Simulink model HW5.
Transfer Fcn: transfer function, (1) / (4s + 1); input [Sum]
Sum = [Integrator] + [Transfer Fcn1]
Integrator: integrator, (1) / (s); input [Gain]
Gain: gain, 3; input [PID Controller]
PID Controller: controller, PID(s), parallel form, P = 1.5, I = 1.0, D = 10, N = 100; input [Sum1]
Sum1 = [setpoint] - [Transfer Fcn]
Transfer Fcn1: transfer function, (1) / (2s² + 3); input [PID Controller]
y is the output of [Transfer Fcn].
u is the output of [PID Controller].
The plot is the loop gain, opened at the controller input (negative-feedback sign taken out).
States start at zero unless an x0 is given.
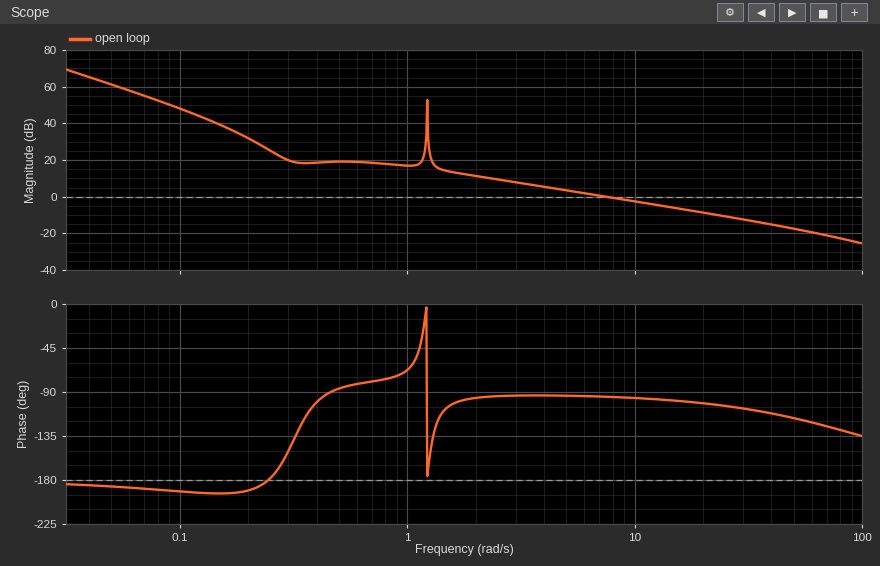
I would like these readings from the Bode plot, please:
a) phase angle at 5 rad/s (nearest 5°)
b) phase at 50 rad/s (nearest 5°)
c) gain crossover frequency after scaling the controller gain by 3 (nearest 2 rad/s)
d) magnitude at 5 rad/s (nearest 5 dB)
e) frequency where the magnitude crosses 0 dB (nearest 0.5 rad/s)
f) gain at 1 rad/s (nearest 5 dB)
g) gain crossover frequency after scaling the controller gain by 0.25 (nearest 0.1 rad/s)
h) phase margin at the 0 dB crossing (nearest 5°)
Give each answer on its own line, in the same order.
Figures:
-95°
-115°
22 rad/s
5 dB
7.5 rad/s
15 dB
1.8 rad/s
85°
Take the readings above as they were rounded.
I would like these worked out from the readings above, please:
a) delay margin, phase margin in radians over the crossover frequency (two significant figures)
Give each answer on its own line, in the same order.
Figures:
0.20 s
